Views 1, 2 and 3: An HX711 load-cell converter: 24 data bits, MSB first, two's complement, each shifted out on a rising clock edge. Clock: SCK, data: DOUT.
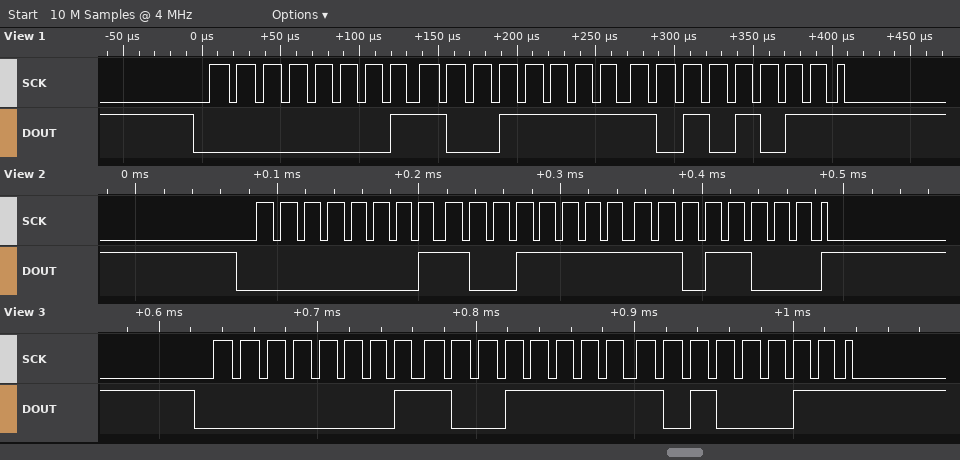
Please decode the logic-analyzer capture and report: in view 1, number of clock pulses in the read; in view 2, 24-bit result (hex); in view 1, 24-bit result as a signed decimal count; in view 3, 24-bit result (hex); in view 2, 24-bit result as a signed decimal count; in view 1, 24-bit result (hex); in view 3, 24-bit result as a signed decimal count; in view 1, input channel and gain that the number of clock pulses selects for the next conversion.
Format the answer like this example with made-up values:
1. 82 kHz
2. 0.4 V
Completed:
1. 25
2. 0x019FD8
3. 106411
4. 0x019FA3
5. 106456
6. 0x019FAB
7. 106403
8. channel A, gain 128
